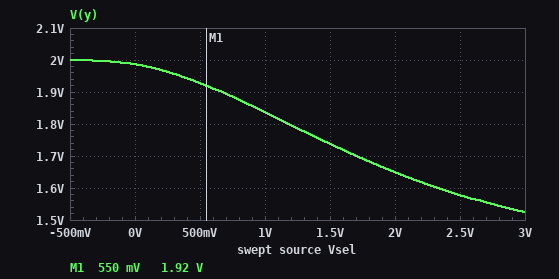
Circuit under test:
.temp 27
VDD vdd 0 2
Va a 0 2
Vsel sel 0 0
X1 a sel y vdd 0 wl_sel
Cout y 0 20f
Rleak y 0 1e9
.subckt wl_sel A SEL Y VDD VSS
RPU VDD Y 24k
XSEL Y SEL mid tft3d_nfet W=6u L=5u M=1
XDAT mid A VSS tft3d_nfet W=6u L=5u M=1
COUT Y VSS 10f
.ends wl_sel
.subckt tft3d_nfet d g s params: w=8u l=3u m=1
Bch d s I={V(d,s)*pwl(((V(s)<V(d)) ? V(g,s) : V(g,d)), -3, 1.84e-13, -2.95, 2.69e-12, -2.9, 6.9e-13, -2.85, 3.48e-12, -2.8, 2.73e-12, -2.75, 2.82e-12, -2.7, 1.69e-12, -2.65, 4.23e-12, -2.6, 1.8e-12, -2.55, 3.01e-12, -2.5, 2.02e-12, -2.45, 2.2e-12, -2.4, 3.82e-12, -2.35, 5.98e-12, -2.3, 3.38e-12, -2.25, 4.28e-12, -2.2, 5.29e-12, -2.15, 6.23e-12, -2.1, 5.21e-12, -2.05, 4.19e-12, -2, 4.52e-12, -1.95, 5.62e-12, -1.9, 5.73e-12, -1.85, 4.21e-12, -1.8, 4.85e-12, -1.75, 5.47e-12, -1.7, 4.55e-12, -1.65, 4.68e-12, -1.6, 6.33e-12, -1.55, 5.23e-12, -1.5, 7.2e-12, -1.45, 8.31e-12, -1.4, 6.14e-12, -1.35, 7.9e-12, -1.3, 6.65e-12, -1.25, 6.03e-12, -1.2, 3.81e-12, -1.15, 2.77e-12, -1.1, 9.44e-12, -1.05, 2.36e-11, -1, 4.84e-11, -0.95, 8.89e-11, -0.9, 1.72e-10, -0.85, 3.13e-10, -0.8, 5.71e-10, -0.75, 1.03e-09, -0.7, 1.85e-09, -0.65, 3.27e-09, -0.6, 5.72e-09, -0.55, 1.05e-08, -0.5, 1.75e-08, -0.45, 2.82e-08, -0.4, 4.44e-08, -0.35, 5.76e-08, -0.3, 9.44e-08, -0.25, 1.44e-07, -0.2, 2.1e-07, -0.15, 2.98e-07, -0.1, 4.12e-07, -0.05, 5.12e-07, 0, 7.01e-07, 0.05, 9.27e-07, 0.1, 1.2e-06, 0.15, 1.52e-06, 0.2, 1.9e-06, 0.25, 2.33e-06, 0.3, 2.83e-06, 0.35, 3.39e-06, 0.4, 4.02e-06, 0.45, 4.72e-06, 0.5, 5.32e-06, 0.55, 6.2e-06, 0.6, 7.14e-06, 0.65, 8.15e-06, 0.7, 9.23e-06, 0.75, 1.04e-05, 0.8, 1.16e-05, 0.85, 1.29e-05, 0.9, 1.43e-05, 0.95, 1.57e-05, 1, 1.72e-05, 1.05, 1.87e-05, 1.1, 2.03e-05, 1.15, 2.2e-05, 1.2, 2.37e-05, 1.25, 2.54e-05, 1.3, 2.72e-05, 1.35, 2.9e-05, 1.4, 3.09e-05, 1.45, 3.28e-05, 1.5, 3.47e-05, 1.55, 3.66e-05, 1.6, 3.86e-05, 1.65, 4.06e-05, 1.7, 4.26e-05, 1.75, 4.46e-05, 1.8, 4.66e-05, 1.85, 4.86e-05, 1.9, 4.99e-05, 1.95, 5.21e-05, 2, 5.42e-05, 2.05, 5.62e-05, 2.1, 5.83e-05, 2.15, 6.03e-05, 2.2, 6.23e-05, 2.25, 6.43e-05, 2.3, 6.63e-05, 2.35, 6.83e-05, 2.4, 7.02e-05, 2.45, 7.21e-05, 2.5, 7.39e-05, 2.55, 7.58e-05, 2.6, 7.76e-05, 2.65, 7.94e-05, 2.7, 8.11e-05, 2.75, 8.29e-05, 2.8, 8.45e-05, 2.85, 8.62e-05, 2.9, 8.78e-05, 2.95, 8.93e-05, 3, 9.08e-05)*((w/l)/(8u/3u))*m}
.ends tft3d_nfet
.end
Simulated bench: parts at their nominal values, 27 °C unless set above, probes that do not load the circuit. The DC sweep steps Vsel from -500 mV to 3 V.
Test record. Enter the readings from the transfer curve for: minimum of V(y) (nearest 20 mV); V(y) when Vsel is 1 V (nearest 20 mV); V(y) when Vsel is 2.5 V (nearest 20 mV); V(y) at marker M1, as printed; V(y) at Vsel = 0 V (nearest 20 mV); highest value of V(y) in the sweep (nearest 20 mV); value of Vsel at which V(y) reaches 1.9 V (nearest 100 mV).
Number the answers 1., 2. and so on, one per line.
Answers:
1. 1.52 V
2. 1.84 V
3. 1.58 V
4. 1.92 V
5. 1.98 V
6. 2.00 V
7. 700 mV
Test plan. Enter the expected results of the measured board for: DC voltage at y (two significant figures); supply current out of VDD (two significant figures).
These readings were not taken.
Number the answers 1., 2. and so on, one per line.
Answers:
1. 2.0 V
2. 550 nA
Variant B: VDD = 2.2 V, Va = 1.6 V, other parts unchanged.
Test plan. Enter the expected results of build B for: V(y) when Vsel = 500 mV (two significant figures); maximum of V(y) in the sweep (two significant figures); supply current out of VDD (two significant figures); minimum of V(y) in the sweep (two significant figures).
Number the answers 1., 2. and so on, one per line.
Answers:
1. 2.1 V
2. 2.2 V
3. 560 nA
4. 1.8 V
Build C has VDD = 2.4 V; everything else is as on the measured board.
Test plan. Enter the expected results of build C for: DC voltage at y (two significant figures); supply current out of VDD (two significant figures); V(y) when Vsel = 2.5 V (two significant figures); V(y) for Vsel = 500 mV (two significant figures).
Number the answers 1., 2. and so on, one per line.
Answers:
1. 2.4 V
2. 640 nA
3. 1.9 V
4. 2.3 V
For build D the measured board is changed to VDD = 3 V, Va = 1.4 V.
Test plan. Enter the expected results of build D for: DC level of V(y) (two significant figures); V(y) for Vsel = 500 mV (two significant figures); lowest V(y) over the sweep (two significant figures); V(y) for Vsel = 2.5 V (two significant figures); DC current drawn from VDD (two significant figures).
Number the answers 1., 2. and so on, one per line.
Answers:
1. 3.0 V
2. 2.9 V
3. 2.5 V
4. 2.6 V
5. 680 nA
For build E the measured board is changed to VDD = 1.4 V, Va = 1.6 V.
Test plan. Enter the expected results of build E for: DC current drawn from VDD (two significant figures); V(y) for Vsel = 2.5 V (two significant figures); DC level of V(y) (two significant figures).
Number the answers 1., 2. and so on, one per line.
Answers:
1. 380 nA
2. 1.1 V
3. 1.4 V
